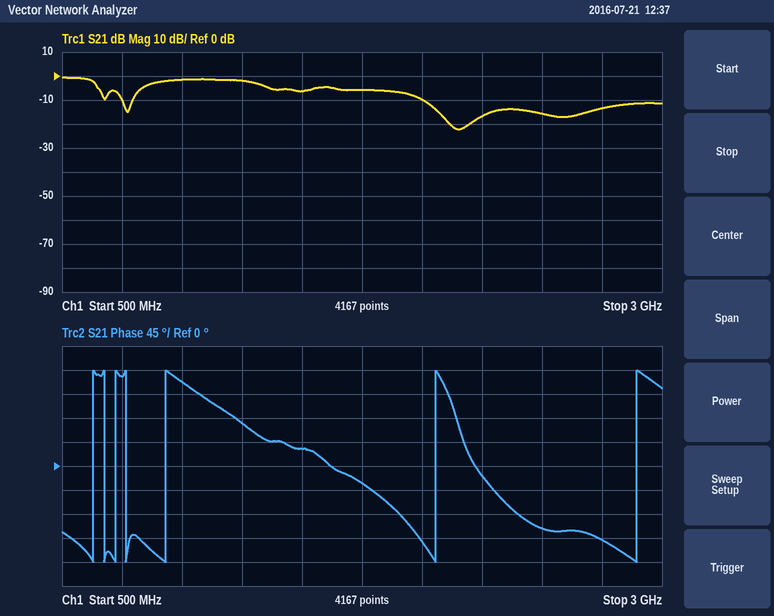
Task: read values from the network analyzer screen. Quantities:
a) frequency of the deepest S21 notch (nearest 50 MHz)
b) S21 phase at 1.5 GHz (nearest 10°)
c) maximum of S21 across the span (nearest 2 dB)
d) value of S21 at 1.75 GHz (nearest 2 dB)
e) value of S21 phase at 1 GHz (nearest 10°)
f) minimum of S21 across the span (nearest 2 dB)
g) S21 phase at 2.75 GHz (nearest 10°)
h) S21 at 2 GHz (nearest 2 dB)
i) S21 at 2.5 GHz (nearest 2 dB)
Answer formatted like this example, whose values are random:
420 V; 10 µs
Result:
2.15 GHz; 30°; 0 dB; -6 dB; 160°; -22 dB; -140°; -10 dB; -16 dB
